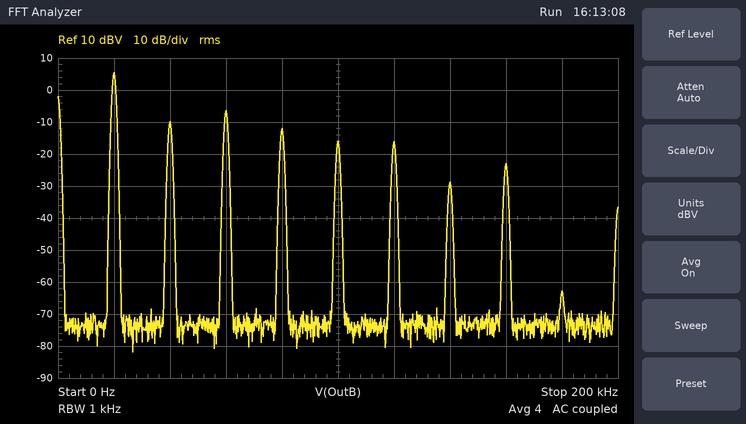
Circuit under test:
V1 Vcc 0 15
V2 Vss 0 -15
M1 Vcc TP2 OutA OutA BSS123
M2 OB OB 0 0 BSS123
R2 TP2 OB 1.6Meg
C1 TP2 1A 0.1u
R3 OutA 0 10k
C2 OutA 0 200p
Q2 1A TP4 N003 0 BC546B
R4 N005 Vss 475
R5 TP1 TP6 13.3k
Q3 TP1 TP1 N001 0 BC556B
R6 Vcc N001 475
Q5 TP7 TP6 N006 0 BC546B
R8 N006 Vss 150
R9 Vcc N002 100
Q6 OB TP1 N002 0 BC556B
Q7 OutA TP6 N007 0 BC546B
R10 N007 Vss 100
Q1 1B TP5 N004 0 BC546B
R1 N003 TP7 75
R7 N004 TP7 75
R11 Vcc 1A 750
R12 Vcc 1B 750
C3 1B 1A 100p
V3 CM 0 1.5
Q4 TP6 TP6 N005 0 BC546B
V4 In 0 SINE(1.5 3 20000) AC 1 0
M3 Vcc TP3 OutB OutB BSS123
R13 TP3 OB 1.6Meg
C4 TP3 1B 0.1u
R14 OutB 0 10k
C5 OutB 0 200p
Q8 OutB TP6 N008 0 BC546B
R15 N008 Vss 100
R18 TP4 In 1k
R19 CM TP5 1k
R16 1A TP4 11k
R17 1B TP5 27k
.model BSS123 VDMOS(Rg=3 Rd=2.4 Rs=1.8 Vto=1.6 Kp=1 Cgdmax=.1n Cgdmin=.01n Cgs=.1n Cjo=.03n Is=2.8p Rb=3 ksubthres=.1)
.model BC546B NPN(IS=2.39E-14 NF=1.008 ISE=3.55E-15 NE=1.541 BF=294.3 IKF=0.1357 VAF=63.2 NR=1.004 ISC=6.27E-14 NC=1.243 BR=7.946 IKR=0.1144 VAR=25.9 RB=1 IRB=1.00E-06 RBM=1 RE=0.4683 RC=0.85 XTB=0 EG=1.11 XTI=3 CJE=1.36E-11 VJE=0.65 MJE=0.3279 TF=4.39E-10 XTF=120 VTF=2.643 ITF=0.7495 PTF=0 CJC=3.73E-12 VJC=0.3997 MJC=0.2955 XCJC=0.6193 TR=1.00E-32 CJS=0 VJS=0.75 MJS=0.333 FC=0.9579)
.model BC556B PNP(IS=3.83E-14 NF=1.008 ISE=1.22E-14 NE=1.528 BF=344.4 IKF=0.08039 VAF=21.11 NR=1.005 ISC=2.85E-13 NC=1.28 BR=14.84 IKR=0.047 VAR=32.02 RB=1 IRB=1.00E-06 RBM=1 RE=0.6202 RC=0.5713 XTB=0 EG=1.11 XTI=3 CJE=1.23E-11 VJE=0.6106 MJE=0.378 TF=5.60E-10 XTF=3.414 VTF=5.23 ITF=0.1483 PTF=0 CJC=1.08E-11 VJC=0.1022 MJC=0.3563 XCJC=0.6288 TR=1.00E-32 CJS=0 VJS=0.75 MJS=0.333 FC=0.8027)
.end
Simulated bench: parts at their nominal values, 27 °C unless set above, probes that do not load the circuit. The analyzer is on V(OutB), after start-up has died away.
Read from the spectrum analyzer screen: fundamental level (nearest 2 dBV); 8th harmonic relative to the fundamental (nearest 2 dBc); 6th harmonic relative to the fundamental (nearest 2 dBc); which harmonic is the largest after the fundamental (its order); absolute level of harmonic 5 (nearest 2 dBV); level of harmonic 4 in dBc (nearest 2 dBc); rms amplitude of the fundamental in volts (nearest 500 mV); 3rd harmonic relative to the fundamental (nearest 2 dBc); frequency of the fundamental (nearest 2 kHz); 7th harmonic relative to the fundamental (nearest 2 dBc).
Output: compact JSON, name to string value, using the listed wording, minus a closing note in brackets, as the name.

{"fundamental level": "6 dBV", "8th harmonic relative to the fundamental": "-28 dBc", "6th harmonic relative to the fundamental": "-22 dBc", "which harmonic is the largest after the fundamental": "3", "absolute level of harmonic 5": "-16 dBV", "level of harmonic 4 in dBc": "-18 dBc", "rms amplitude of the fundamental in volts": "2.0 V", "3rd harmonic relative to the fundamental": "-12 dBc", "frequency of the fundamental": "20 kHz", "7th harmonic relative to the fundamental": "-34 dBc"}
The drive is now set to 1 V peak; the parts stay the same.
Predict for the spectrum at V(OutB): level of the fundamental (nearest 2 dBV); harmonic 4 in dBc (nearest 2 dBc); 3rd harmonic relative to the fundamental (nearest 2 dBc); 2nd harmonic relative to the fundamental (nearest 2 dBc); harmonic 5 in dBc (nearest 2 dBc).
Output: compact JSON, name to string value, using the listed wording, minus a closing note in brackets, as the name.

{"level of the fundamental": "2 dBV", "harmonic 4 in dBc": "-34 dBc", "3rd harmonic relative to the fundamental": "-22 dBc", "2nd harmonic relative to the fundamental": "-12 dBc", "harmonic 5 in dBc": "-30 dBc"}
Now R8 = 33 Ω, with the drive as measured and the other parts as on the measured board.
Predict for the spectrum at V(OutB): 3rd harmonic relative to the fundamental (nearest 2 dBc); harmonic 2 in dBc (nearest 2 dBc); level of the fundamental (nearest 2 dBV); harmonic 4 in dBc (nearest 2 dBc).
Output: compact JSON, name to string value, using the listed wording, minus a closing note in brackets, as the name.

{"3rd harmonic relative to the fundamental": "-18 dBc", "harmonic 2 in dBc": "-20 dBc", "level of the fundamental": "12 dBV", "harmonic 4 in dBc": "-30 dBc"}
